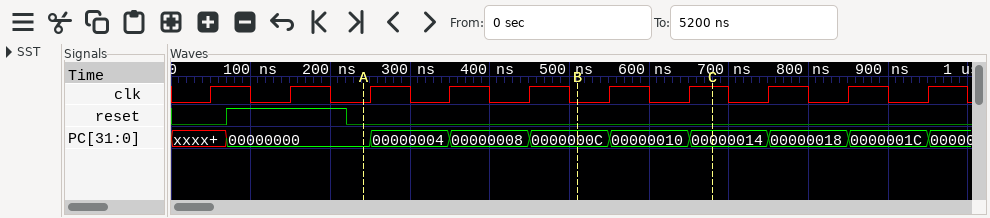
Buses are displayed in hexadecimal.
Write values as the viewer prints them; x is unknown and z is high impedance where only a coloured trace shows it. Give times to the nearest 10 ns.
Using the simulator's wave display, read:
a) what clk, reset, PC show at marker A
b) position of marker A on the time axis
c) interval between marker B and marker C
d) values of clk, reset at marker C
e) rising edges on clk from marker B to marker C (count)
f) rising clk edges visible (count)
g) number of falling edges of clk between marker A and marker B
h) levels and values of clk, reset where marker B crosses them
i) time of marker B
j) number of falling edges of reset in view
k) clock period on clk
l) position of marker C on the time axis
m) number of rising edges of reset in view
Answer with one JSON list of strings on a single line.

["clk=0, reset=0, PC=00000000", "240 ns", "170 ns", "clk=1, reset=0", "2", "10", "3", "clk=0, reset=0", "510 ns", "1", "100 ns", "680 ns", "1"]
